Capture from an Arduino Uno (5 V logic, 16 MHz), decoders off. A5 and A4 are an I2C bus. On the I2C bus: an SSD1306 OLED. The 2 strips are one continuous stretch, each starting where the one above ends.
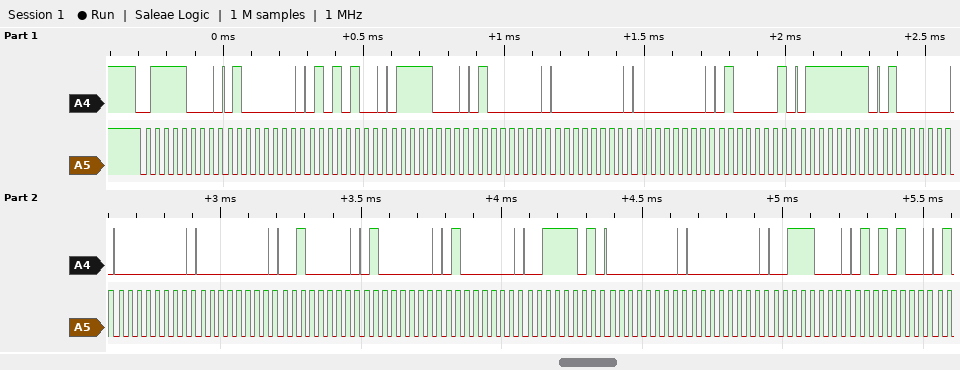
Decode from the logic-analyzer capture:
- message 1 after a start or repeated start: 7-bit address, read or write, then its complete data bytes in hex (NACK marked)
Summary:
0x3C write: 40 54 78 40 00 00 41 7F 40 00 00 20 40 40 3D 00 00 38 54
